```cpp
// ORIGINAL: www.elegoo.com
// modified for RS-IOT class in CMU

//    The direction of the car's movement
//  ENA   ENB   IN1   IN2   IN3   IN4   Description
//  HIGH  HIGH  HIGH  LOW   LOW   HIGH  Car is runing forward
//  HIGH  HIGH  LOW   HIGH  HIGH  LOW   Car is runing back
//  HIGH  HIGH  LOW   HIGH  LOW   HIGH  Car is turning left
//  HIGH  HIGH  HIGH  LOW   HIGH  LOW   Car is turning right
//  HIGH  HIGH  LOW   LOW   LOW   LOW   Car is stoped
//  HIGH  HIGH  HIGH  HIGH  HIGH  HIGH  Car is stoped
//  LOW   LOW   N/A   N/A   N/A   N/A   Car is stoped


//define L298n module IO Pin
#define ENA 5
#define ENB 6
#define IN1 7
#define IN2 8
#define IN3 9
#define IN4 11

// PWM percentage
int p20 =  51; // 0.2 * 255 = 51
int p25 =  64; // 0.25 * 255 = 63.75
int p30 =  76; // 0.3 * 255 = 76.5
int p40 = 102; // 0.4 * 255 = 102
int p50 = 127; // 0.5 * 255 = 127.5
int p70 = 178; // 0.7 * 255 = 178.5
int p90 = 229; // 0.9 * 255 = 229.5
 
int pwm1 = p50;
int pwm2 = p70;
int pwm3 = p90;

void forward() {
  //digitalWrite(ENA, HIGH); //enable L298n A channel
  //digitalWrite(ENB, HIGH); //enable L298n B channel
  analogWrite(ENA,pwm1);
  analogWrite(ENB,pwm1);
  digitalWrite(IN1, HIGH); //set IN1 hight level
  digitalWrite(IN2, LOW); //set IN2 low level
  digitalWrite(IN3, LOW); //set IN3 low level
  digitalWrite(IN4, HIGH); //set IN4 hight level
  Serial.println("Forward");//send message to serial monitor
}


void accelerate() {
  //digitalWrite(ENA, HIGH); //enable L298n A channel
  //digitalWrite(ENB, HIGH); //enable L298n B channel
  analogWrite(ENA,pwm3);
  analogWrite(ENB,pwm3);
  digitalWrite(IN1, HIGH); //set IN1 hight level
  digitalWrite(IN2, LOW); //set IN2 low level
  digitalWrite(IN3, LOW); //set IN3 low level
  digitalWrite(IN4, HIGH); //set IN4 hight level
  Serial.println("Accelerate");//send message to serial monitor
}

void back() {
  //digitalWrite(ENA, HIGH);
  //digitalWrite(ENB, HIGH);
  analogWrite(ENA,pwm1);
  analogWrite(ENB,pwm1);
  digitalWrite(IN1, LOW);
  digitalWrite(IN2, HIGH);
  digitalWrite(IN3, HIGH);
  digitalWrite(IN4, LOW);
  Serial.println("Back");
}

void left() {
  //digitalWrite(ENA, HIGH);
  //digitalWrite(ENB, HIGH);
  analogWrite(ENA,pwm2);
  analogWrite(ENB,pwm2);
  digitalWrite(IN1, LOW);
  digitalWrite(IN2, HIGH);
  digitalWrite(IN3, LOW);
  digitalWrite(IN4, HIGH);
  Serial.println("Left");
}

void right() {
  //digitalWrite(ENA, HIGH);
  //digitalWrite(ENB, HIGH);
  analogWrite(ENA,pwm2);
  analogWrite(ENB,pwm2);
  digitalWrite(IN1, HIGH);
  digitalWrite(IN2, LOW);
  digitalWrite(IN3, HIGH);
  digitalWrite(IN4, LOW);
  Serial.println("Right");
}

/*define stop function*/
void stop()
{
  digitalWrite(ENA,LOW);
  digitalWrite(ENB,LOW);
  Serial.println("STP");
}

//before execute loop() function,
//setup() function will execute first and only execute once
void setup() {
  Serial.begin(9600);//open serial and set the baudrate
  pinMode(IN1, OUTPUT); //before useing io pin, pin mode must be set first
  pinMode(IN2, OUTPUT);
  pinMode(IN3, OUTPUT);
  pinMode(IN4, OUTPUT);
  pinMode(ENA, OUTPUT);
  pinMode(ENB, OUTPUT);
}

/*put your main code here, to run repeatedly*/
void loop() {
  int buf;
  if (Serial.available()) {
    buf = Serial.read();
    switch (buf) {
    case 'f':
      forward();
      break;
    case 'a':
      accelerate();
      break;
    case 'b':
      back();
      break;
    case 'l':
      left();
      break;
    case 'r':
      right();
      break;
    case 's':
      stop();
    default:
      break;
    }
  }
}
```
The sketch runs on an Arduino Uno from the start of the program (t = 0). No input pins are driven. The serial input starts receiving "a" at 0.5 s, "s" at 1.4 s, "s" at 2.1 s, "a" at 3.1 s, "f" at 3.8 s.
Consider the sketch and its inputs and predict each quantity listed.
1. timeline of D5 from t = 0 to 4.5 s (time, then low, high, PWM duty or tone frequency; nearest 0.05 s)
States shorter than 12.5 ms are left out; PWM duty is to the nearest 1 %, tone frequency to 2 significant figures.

0 s low; 0.5 s PWM 90 %; 1.4 s low; 3.1 s PWM 90 %; 3.8 s PWM 50 %
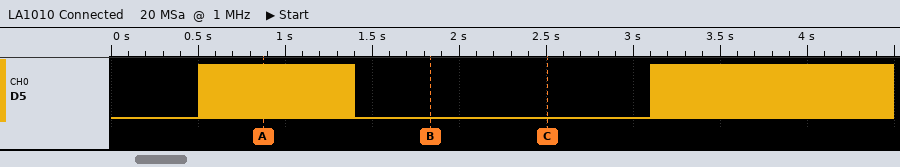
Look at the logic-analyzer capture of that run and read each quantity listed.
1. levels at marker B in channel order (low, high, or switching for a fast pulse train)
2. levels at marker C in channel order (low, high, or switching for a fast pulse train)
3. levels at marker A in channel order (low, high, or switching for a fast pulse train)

D5 low
D5 low
D5 switching
